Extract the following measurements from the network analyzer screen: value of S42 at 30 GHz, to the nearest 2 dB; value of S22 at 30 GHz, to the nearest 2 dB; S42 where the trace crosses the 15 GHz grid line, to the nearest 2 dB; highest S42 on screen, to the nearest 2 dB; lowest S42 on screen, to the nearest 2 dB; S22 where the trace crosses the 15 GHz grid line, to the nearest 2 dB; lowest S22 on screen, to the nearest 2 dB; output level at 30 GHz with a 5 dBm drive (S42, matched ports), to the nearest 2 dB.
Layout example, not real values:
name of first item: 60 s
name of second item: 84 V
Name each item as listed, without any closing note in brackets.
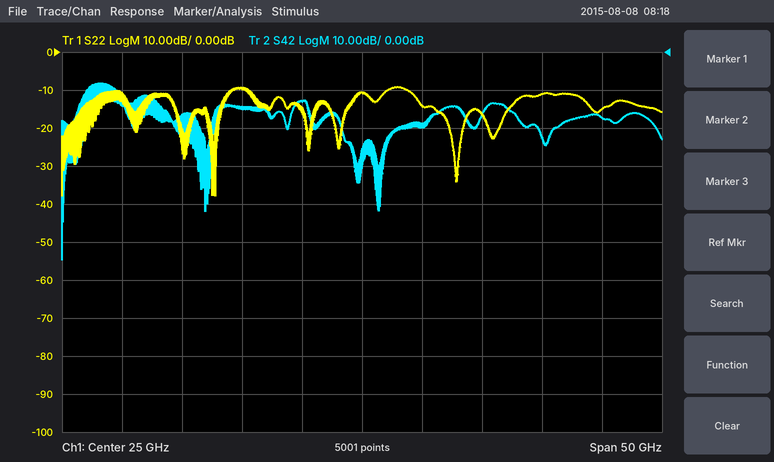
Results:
value of S42 at 30 GHz, to the nearest 2 dB: -20 dB
value of S22 at 30 GHz, to the nearest 2 dB: -14 dB
S42 where the trace crosses the 15 GHz grid line, to the nearest 2 dB: -14 dB
highest S42 on screen, to the nearest 2 dB: -8 dB
lowest S42 on screen, to the nearest 2 dB: -54 dB
S22 where the trace crosses the 15 GHz grid line, to the nearest 2 dB: -10 dB
lowest S22 on screen, to the nearest 2 dB: -38 dB
output level at 30 GHz with a 5 dBm drive (S42, matched ports), to the nearest 2 dB: -14 dBm
